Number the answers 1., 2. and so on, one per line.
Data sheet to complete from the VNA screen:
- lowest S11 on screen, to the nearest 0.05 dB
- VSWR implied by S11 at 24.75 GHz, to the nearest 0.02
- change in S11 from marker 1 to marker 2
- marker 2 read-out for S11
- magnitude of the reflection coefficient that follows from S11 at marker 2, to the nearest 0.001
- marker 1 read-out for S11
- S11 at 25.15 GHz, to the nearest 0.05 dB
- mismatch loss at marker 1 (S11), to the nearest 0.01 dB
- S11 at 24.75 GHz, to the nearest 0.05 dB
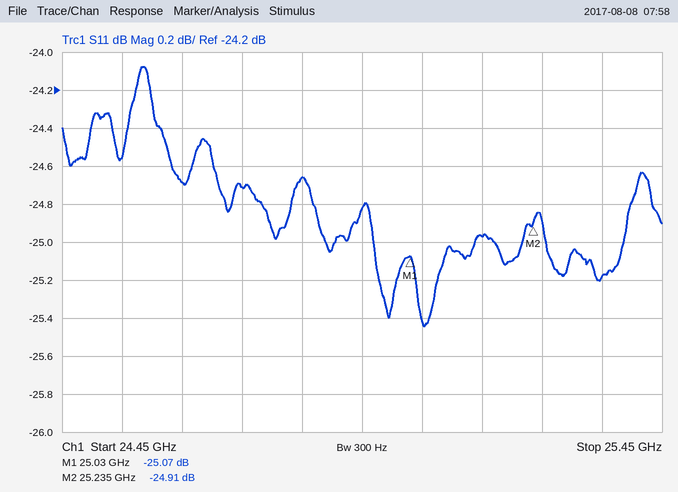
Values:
1. -25.45 dB
2. 1.12
3. 0.16 dB
4. -24.91 dB
5. 0.057
6. -25.07 dB
7. -24.95 dB
8. 0.01 dB
9. -24.70 dB
